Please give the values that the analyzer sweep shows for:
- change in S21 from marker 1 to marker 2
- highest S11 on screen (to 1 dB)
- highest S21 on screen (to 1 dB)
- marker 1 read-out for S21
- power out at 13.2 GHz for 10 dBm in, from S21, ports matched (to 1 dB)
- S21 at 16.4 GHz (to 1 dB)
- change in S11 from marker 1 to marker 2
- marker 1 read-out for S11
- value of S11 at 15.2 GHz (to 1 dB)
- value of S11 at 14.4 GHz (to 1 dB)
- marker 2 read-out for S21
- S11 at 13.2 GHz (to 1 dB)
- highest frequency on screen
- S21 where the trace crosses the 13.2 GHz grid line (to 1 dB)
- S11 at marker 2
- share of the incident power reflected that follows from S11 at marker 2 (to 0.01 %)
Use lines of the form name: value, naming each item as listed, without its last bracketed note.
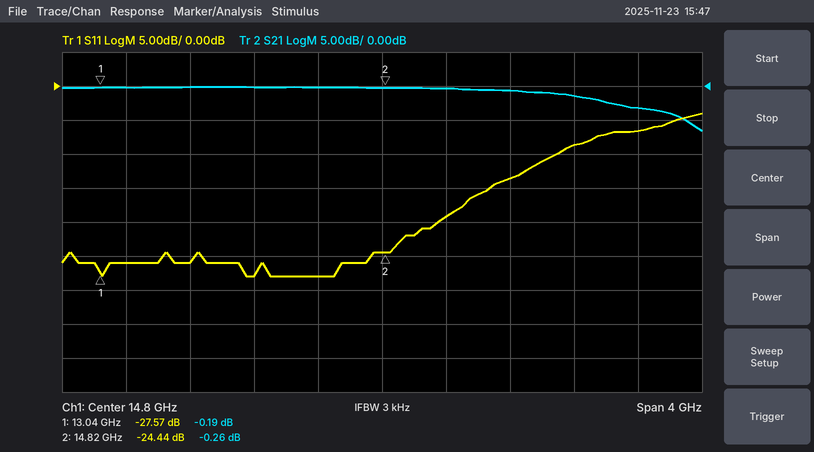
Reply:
change in S21 from marker 1 to marker 2: -0.07 dB
highest S11 on screen: -4 dB
highest S21 on screen: 0 dB
marker 1 read-out for S21: -0.19 dB
power out at 13.2 GHz for 10 dBm in, from S21, ports matched: 10 dBm
S21 at 16.4 GHz: -3 dB
change in S11 from marker 1 to marker 2: 3.13 dB
marker 1 read-out for S11: -27.57 dB
value of S11 at 15.2 GHz: -19 dB
value of S11 at 14.4 GHz: -28 dB
marker 2 read-out for S21: -0.26 dB
S11 at 13.2 GHz: -26 dB
highest frequency on screen: 16.8 GHz
S21 where the trace crosses the 13.2 GHz grid line: 0 dB
S11 at marker 2: -24.44 dB
share of the incident power reflected that follows from S11 at marker 2: 0.36 %
